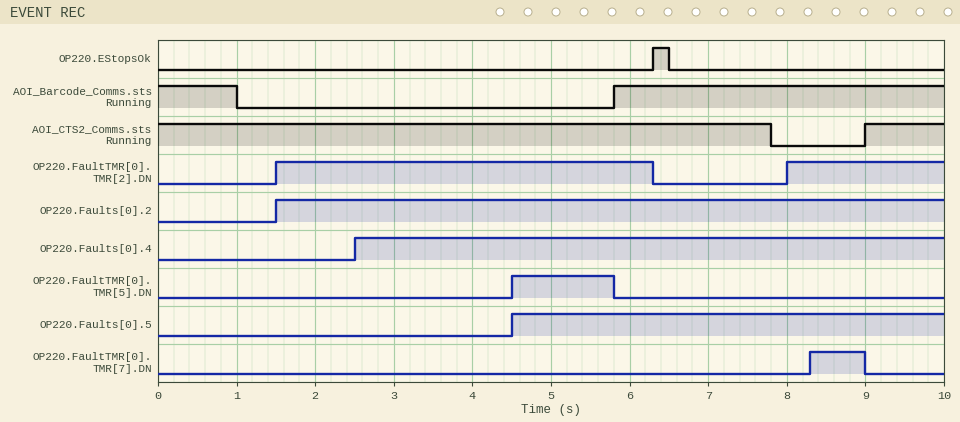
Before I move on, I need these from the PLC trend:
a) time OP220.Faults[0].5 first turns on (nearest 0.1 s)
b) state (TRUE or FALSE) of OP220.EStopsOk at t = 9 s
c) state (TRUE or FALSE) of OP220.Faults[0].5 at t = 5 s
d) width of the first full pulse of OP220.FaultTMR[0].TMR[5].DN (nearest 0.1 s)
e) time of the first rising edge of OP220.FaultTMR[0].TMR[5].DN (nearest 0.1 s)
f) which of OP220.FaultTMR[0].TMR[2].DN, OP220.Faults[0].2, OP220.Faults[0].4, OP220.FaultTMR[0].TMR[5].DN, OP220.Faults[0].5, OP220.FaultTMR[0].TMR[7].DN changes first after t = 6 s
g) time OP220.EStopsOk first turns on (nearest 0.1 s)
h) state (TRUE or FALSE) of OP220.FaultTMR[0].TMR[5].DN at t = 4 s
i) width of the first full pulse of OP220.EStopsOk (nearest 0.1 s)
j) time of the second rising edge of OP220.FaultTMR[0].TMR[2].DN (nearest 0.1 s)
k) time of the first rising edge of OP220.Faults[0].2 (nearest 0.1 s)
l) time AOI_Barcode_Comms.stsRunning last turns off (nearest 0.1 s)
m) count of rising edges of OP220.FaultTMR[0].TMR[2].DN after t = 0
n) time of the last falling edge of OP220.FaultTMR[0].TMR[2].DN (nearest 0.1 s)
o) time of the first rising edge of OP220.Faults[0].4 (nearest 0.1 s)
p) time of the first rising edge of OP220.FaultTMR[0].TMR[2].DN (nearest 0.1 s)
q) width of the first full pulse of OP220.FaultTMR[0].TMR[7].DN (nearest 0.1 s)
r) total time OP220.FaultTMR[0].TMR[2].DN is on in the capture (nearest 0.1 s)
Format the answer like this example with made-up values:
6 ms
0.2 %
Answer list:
4.5 s
FALSE
TRUE
1.3 s
4.5 s
OP220.FaultTMR[0].TMR[2].DN
6.3 s
FALSE
0.2 s
8.0 s
1.5 s
1.0 s
2
6.3 s
2.5 s
1.5 s
0.7 s
6.8 s
